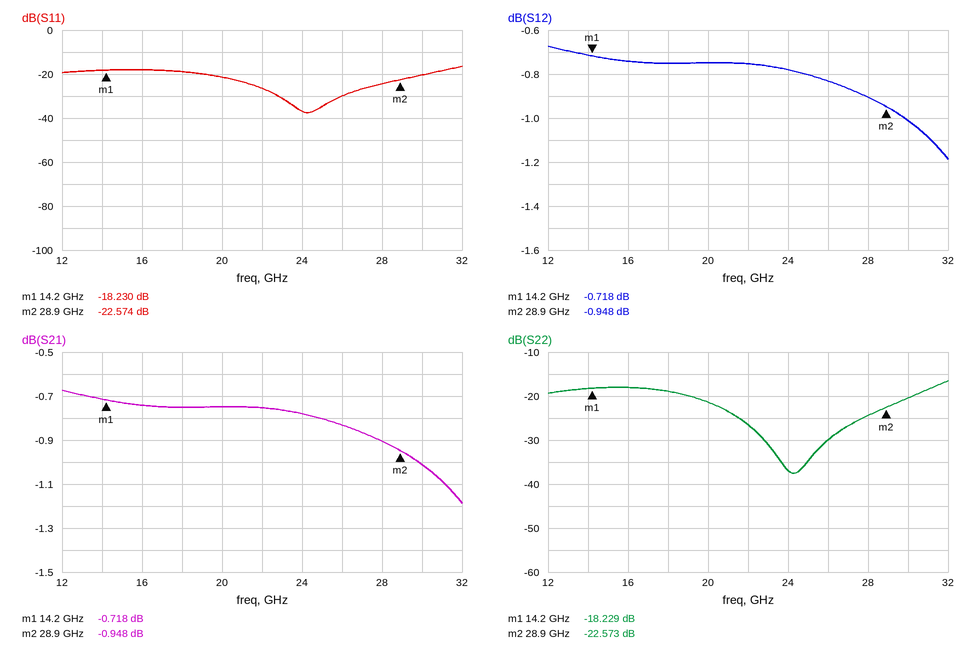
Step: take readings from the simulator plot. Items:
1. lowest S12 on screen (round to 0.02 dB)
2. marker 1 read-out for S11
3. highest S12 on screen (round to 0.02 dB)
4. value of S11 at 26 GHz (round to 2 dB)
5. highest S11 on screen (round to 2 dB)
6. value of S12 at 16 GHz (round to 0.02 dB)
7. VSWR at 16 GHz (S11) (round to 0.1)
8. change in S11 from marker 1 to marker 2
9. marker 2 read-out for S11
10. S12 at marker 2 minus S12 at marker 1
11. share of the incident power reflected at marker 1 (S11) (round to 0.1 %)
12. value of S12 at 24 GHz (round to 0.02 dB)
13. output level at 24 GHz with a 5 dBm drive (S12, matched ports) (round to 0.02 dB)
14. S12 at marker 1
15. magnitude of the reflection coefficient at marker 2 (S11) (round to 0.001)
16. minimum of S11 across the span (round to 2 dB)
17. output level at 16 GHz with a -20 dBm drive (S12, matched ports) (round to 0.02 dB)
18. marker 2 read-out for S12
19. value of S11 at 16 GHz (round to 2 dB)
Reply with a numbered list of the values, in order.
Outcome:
1. -1.18 dB
2. -18.230 dB
3. -0.68 dB
4. -30 dB
5. -16 dB
6. -0.74 dB
7. 1.3
8. -4.344 dB
9. -22.574 dB
10. -0.230 dB
11. 1.5 %
12. -0.78 dB
13. 4.22 dBm
14. -0.718 dB
15. 0.074
16. -38 dB
17. -20.74 dBm
18. -0.948 dB
19. -18 dB
